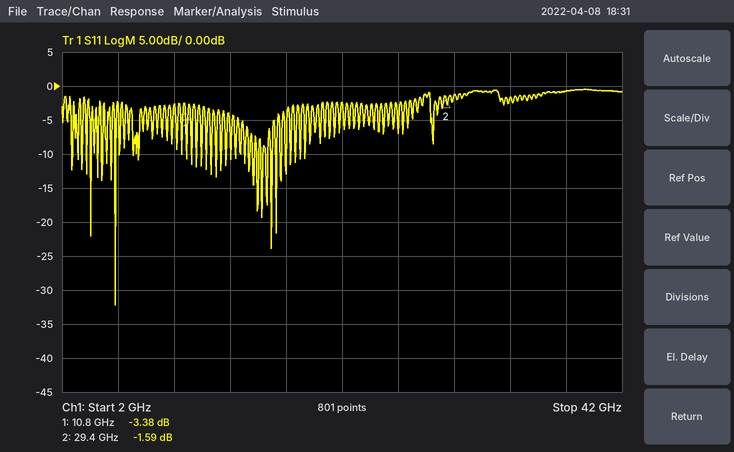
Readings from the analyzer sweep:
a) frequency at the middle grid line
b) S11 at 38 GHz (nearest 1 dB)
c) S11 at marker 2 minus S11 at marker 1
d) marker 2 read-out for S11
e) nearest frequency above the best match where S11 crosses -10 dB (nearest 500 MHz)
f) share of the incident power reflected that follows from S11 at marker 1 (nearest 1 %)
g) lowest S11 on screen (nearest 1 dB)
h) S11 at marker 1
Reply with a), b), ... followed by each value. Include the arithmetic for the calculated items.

a) 22 GHz
b) -1 dB
c) -1.59 − (-3.38) = 1.79 dB
d) -1.59 dB
e) 6.0 GHz
f) 10^(-3.38/10) ≈ 46 %
g) -32 dB
h) -3.38 dB
